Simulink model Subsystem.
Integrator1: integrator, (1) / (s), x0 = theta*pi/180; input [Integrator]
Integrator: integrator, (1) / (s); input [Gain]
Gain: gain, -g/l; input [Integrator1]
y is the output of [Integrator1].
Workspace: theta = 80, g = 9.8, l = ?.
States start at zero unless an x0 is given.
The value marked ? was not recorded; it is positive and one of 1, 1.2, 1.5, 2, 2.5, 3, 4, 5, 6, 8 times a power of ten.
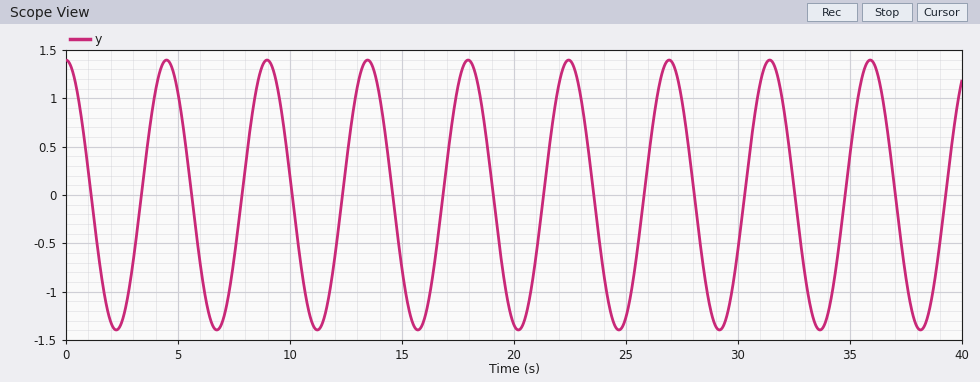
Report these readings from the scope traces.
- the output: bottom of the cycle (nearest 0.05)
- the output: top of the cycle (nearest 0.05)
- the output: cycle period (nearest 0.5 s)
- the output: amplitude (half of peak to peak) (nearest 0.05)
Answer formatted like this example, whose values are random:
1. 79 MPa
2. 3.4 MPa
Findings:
1. -1.40
2. 1.40
3. 4.5 s
4. 1.40
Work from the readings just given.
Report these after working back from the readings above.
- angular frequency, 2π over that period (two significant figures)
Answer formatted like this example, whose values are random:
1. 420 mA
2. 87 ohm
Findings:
1. 1.4 rad/s
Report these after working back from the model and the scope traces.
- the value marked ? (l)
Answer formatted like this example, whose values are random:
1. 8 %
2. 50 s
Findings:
1. 5
